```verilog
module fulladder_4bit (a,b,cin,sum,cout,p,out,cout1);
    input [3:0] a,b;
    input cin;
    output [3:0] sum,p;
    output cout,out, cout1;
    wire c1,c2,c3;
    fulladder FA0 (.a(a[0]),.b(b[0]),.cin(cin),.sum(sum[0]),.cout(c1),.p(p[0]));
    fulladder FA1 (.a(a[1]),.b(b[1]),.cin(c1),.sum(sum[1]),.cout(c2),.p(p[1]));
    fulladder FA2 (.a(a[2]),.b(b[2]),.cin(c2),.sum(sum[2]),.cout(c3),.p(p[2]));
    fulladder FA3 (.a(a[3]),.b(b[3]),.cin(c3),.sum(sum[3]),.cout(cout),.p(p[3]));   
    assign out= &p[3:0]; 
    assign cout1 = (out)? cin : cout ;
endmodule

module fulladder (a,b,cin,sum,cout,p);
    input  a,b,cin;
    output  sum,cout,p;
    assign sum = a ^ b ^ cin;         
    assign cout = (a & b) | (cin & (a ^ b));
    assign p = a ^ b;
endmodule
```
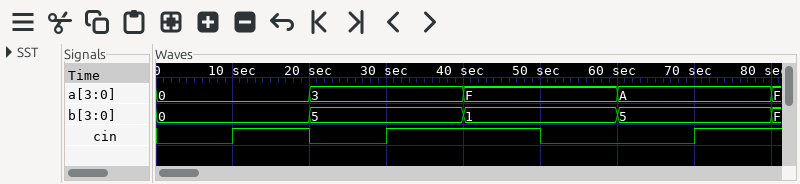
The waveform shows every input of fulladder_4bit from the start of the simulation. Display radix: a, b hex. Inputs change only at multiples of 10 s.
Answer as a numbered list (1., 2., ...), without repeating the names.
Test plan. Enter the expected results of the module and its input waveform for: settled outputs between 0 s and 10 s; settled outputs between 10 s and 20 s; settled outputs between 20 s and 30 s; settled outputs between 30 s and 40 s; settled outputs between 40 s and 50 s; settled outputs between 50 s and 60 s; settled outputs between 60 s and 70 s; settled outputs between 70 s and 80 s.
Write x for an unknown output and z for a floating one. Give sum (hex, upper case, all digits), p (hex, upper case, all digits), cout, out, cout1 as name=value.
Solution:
1. sum=0, p=0, cout=0, out=0, cout1=0
2. sum=1, p=0, cout=0, out=0, cout1=0
3. sum=8, p=6, cout=0, out=0, cout1=0
4. sum=9, p=6, cout=0, out=0, cout1=0
5. sum=1, p=E, cout=1, out=0, cout1=1
6. sum=0, p=E, cout=1, out=0, cout1=1
7. sum=F, p=F, cout=0, out=1, cout1=0
8. sum=0, p=F, cout=1, out=1, cout1=1
